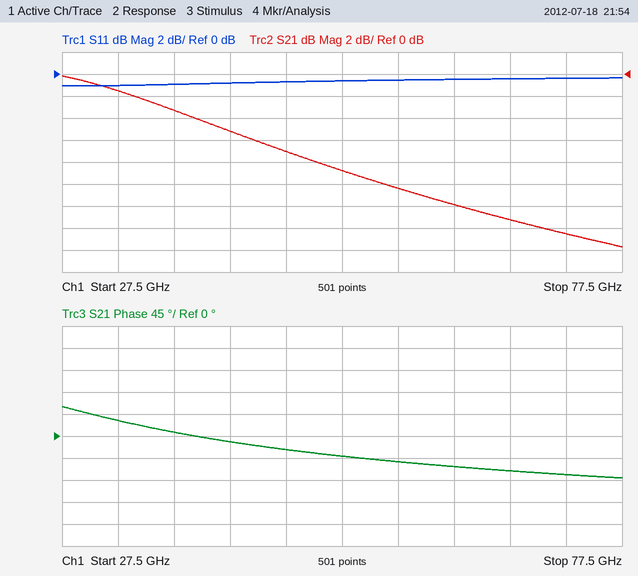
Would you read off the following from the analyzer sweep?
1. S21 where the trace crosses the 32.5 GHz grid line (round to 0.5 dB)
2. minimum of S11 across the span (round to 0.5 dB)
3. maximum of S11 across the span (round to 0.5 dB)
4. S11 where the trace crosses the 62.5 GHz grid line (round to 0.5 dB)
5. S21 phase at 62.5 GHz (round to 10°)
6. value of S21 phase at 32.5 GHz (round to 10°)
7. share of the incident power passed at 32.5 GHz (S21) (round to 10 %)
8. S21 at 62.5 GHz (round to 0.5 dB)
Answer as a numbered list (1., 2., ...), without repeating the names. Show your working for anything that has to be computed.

1. -1.5 dB
2. -1.0 dB
3. -0.5 dB
4. -0.5 dB
5. -60°
6. 30°
7. 10^(-1.5/10) ≈ 70.8 %, so 70 % to the nearest 10 %
8. -12.0 dB
